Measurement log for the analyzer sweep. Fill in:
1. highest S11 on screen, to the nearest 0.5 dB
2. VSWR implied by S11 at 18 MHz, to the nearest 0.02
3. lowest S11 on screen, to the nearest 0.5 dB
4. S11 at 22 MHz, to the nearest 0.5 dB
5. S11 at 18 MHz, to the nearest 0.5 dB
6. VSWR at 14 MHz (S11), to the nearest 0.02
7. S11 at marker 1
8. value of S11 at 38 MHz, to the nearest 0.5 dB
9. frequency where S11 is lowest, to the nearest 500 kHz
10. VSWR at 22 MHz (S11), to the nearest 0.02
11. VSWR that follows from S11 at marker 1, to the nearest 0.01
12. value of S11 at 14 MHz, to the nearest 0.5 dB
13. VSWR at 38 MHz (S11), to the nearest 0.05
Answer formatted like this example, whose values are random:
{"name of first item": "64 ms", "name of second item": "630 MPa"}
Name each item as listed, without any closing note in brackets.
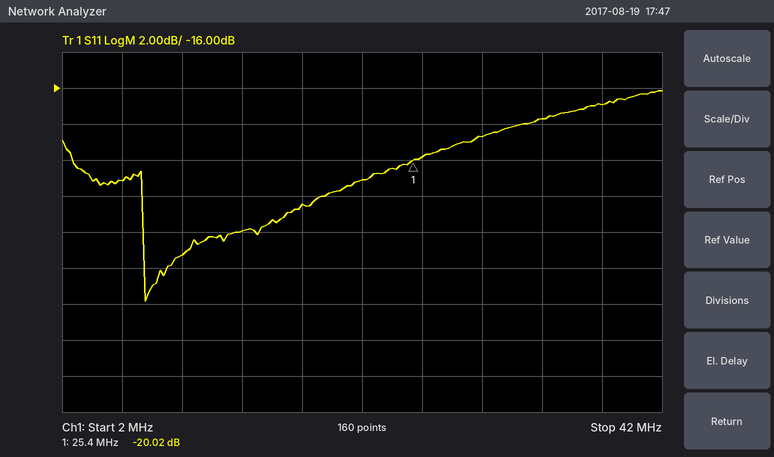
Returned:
{"highest S11 on screen, to the nearest 0.5 dB": "-16.0 dB", "VSWR implied by S11 at 18 MHz, to the nearest 0.02": "1.16", "lowest S11 on screen, to the nearest 0.5 dB": "-28.0 dB", "S11 at 22 MHz, to the nearest 0.5 dB": "-21.0 dB", "S11 at 18 MHz, to the nearest 0.5 dB": "-22.5 dB", "VSWR at 14 MHz (S11), to the nearest 0.02": "1.14", "S11 at marker 1": "-20.02 dB", "value of S11 at 38 MHz, to the nearest 0.5 dB": "-17.0 dB", "frequency where S11 is lowest, to the nearest 500 kHz": "7.5 MHz", "VSWR at 22 MHz (S11), to the nearest 0.02": "1.20", "VSWR that follows from S11 at marker 1, to the nearest 0.01": "1.22", "value of S11 at 14 MHz, to the nearest 0.5 dB": "-24.0 dB", "VSWR at 38 MHz (S11), to the nearest 0.05": "1.35"}
